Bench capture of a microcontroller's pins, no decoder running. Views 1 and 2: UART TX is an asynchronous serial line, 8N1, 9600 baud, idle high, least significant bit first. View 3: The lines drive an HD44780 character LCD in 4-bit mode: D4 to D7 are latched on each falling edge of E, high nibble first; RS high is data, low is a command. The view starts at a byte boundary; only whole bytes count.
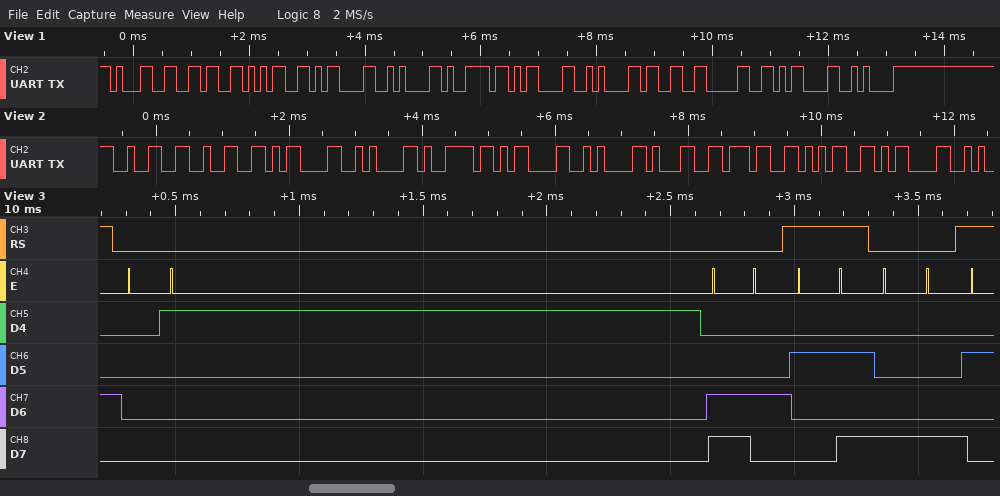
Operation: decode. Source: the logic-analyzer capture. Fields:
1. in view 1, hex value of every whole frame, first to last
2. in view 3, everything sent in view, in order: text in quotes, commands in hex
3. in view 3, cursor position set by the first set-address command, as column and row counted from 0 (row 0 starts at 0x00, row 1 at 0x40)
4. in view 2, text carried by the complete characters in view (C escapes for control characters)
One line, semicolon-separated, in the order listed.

0x31 0x36 0x35 0x0D 0x0A 0x79 0x0D 0x0A 0x33 0x30 0x0D 0x0A; 0x01 0xC4 "*" 0x88; column 4, row 1; "22\r\ny\r\n175\r"
